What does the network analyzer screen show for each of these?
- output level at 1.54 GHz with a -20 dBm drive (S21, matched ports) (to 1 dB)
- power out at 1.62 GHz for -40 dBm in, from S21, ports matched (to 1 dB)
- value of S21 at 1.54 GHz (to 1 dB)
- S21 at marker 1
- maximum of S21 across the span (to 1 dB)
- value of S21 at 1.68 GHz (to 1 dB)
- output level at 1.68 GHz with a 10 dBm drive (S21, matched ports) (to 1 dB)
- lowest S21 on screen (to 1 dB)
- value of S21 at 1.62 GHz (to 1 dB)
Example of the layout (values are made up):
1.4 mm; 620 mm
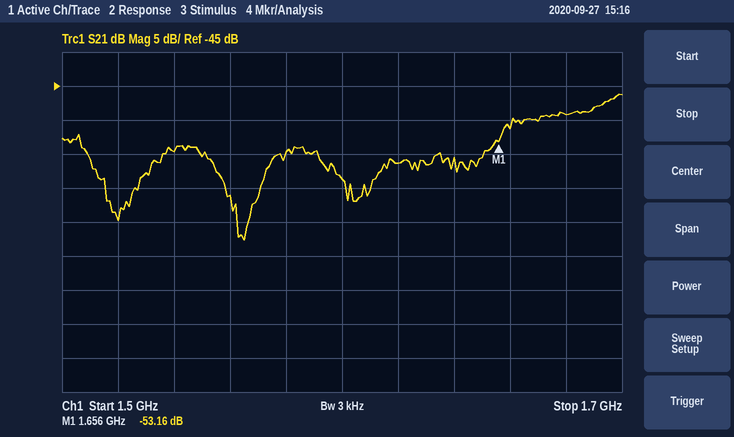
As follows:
-75 dBm; -96 dBm; -55 dB; -53.16 dB; -46 dB; -49 dB; -39 dBm; -68 dB; -56 dB
